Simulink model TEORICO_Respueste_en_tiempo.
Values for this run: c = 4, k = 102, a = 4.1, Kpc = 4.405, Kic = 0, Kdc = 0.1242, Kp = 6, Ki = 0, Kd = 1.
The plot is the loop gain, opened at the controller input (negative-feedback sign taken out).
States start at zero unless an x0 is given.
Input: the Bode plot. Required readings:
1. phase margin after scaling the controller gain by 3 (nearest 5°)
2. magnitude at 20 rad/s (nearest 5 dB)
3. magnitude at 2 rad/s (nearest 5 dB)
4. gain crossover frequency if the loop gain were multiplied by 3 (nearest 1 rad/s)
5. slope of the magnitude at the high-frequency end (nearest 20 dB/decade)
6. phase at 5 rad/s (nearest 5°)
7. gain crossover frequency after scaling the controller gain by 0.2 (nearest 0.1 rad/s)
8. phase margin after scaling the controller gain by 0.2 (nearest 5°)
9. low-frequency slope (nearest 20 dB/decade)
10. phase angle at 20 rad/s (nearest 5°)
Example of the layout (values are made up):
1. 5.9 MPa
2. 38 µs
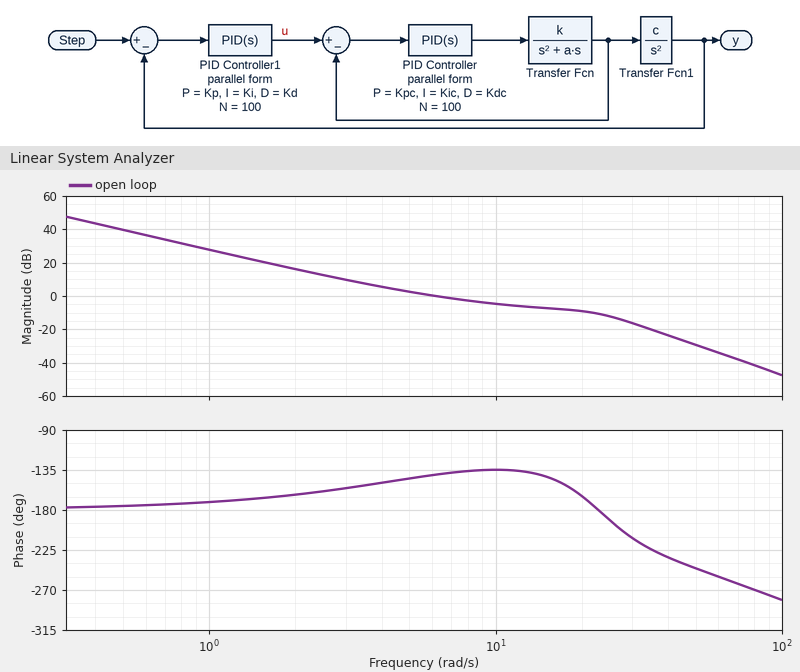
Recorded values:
1. 10°
2. -10 dB
3. 15 dB
4. 21 rad/s
5. -60 dB/decade
6. -145°
7. 2.3 rad/s
8. 20°
9. -40 dB/decade
10. -165°
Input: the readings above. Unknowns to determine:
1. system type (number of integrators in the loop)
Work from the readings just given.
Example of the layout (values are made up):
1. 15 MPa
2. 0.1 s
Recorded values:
1. 2
